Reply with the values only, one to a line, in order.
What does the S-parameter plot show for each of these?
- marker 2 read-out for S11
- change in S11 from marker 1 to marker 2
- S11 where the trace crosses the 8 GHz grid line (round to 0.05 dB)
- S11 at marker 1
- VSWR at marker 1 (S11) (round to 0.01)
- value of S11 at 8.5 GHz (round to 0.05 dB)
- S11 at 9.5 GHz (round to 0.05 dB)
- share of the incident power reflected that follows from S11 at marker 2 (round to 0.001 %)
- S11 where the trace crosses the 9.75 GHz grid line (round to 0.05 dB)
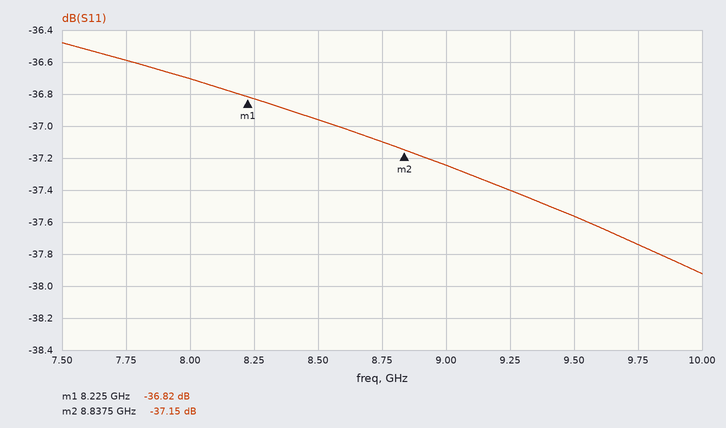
-37.15 dB
-0.33 dB
-36.70 dB
-36.82 dB
1.03
-36.95 dB
-37.55 dB
0.019 %
-37.75 dB
